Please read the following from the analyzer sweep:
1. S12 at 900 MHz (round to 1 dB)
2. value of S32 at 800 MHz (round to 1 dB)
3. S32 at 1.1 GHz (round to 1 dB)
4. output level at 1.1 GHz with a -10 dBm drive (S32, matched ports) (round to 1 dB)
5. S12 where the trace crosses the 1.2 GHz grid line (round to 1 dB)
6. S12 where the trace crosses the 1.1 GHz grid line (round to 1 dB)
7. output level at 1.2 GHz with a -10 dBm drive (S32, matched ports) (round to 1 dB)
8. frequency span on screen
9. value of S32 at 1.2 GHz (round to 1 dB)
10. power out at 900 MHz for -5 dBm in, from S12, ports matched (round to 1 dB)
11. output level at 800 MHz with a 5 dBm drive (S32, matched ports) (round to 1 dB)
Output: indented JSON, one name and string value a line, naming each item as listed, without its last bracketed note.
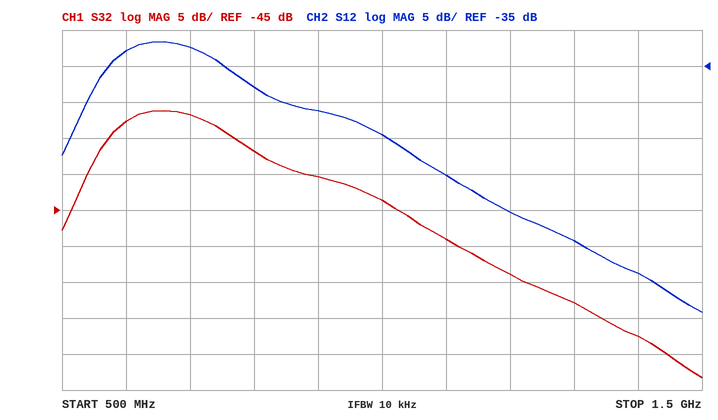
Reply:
{
  "S12 at 900 MHz": "-41 dB",
  "value of S32 at 800 MHz": "-37 dB",
  "S32 at 1.1 GHz": "-49 dB",
  "output level at 1.1 GHz with a -10 dBm drive (S32, matched ports)": "-59 dBm",
  "S12 where the trace crosses the 1.2 GHz grid line": "-55 dB",
  "S12 where the trace crosses the 1.1 GHz grid line": "-50 dB",
  "output level at 1.2 GHz with a -10 dBm drive (S32, matched ports)": "-64 dBm",
  "frequency span on screen": "1 GHz",
  "value of S32 at 1.2 GHz": "-54 dB",
  "power out at 900 MHz for -5 dBm in, from S12, ports matched": "-46 dBm",
  "output level at 800 MHz with a 5 dBm drive (S32, matched ports)": "-32 dBm"
}
